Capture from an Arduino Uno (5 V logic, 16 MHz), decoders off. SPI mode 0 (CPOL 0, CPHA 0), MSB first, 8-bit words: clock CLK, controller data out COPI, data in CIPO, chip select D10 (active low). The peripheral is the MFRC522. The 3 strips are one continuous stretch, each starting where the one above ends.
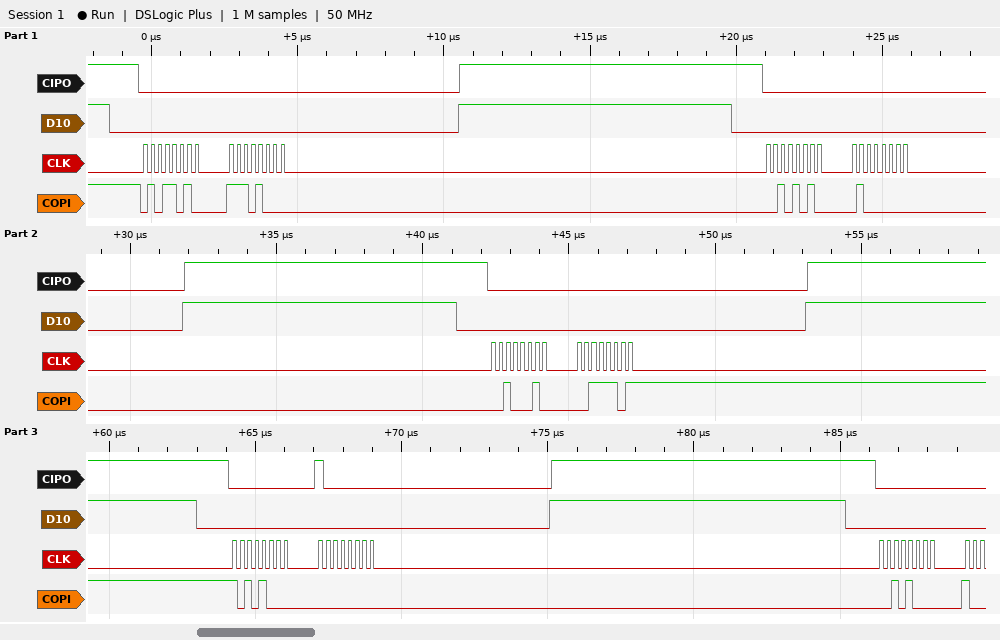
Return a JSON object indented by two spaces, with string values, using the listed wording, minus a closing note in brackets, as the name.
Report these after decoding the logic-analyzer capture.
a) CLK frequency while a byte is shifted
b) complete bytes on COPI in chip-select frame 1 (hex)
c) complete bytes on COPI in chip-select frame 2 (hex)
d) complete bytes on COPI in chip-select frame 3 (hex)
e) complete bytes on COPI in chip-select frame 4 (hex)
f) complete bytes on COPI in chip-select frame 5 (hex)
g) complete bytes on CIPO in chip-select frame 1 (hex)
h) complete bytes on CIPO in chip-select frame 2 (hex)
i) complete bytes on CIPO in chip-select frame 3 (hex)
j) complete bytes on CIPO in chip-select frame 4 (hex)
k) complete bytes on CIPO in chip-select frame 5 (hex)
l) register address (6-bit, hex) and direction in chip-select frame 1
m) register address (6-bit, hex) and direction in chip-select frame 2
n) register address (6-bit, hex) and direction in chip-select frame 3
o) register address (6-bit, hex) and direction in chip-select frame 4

{
  "CLK frequency while a byte is shifted": "4 MHz",
  "complete bytes on COPI in chip-select frame 1": "5A E8",
  "complete bytes on COPI in chip-select frame 2": "2A 40",
  "complete bytes on COPI in chip-select frame 3": "22 3D",
  "complete bytes on COPI in chip-select frame 4": "A8 00",
  "complete bytes on COPI in chip-select frame 5": "28",
  "complete bytes on CIPO in chip-select frame 1": "00 00",
  "complete bytes on CIPO in chip-select frame 2": "00 00",
  "complete bytes on CIPO in chip-select frame 3": "00 00",
  "complete bytes on CIPO in chip-select frame 4": "00 80",
  "complete bytes on CIPO in chip-select frame 5": "00",
  "register address (6-bit, hex) and direction in chip-select frame 1": "0x2D write",
  "register address (6-bit, hex) and direction in chip-select frame 2": "0x15 write",
  "register address (6-bit, hex) and direction in chip-select frame 3": "0x11 write",
  "register address (6-bit, hex) and direction in chip-select frame 4": "0x14 read"
}
